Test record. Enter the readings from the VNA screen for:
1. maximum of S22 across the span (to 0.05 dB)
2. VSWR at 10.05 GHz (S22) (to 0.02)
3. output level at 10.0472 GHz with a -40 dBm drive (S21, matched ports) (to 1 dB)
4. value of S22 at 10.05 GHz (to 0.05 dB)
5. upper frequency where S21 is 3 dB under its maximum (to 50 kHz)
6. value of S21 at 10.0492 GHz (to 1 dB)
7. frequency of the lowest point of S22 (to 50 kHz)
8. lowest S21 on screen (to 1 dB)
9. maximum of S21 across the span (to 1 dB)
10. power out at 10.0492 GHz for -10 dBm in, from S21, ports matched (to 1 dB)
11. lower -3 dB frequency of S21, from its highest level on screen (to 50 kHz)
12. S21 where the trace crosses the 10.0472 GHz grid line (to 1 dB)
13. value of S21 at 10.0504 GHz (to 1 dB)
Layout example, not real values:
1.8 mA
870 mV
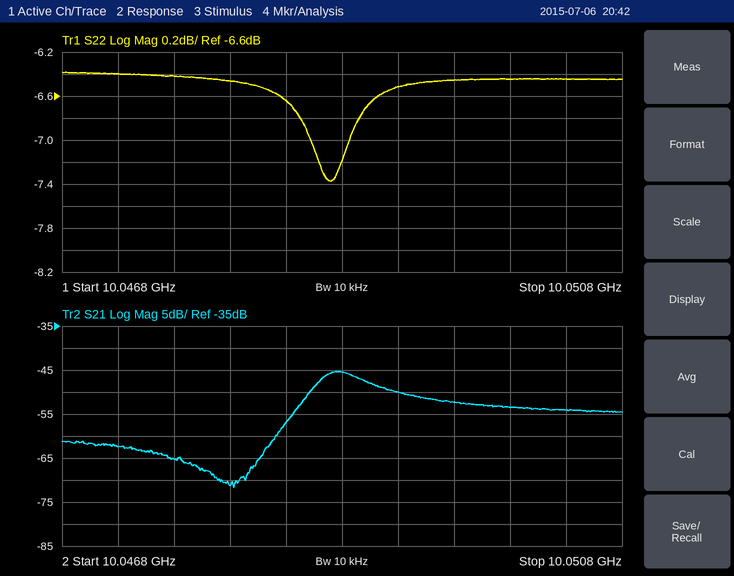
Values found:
-6.40 dB
2.82
-102 dBm
-6.45 dB
10.04905 GHz
-50 dB
10.04870 GHz
-72 dB
-45 dB
-60 dBm
10.04860 GHz
-62 dB
-54 dB
